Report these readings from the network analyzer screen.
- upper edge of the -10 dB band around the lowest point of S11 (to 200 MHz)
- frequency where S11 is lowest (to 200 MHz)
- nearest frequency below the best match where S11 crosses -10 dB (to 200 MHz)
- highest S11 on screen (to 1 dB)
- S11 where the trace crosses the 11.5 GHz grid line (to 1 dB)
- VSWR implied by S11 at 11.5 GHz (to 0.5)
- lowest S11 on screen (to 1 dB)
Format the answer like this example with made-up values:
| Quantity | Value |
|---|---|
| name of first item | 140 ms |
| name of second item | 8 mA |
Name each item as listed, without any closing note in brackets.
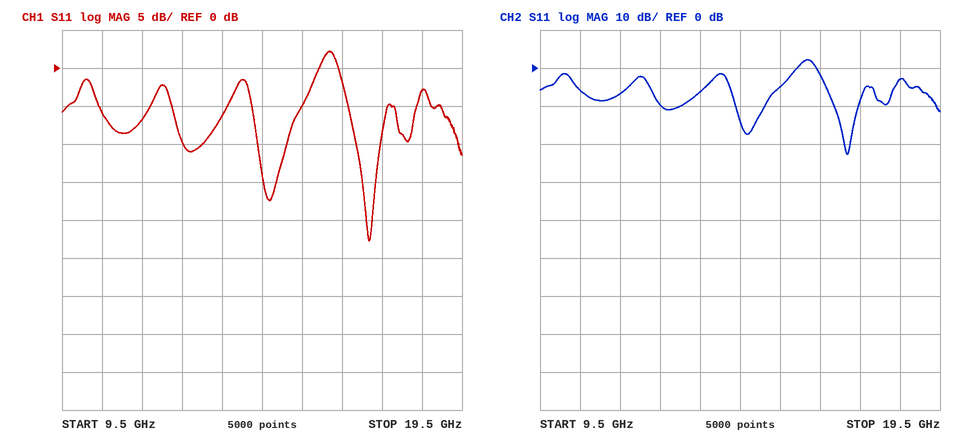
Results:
| Quantity | Value |
|---|---|
| upper edge of the -10 dB band around the lowest point of S11 | 17.4 GHz |
| frequency where S11 is lowest | 17.2 GHz |
| nearest frequency below the best match where S11 crosses -10 dB | 16.8 GHz |
| highest S11 on screen | 2 dB |
| S11 where the trace crosses the 11.5 GHz grid line | -7 dB |
| VSWR implied by S11 at 11.5 GHz | 2.5 |
| lowest S11 on screen | -23 dB |
